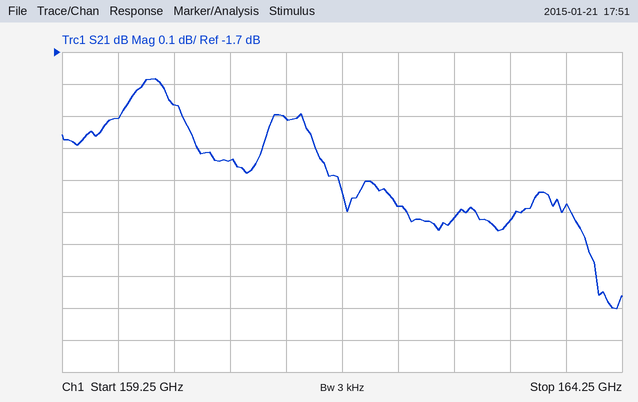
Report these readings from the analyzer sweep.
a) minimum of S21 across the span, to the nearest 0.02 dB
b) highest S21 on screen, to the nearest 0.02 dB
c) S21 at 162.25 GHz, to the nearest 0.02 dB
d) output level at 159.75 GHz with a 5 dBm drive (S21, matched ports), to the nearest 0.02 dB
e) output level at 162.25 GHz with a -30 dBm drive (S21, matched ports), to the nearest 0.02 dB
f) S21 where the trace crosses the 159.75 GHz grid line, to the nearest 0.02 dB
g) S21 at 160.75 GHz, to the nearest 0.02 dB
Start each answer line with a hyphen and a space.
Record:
- -2.50 dB
- -1.78 dB
- -2.18 dB
- 3.10 dBm
- -32.18 dBm
- -1.90 dB
- -2.04 dB
